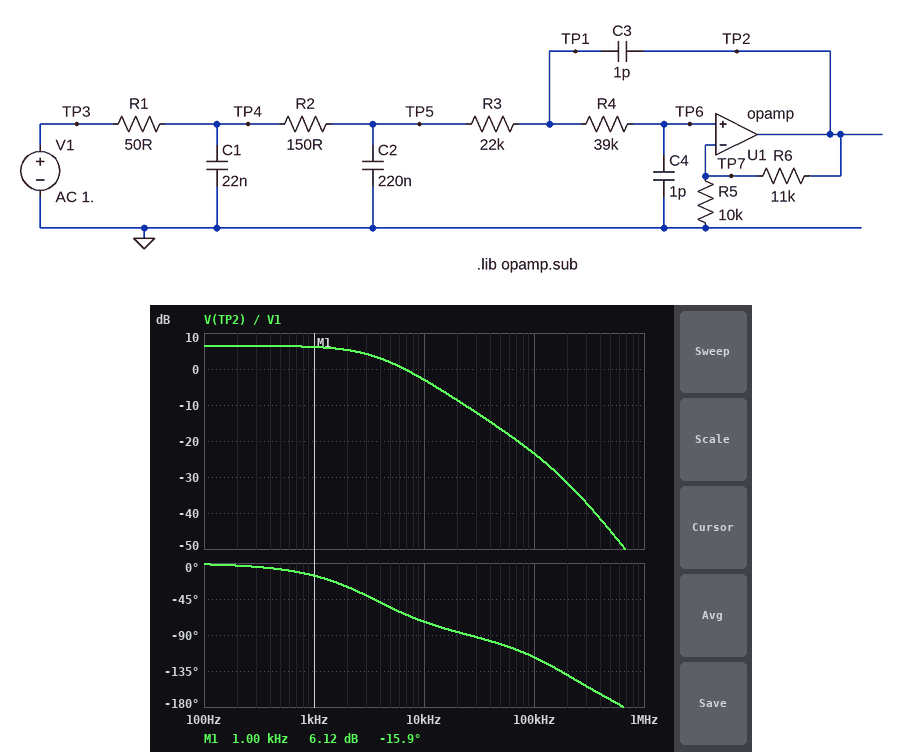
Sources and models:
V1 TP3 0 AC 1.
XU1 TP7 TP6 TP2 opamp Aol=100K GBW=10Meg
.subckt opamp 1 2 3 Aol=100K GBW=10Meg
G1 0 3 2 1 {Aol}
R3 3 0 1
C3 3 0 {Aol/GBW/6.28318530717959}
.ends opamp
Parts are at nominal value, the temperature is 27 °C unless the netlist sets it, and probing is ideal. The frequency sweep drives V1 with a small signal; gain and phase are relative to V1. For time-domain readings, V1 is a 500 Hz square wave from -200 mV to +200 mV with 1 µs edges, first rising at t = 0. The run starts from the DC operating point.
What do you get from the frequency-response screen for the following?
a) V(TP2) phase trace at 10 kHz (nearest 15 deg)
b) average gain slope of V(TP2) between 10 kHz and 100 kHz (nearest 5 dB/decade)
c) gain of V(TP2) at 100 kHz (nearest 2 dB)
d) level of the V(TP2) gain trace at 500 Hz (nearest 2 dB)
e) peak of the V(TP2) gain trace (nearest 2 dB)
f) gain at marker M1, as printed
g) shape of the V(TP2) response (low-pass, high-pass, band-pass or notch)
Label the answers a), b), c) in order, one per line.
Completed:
a) -75 deg
b) -20 dB/decade
c) -24 dB
d) 6 dB
e) 6 dB
f) 6.12 dB
g) low-pass
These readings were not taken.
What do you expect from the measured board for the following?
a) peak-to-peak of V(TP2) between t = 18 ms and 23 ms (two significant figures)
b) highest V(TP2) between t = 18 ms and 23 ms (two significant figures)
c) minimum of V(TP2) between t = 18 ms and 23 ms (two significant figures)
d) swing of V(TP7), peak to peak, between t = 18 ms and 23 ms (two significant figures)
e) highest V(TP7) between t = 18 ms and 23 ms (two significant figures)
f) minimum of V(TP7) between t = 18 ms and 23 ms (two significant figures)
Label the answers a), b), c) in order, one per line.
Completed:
a) 840 mV
b) 420 mV
c) -420 mV
d) 400 mV
e) 200 mV
f) -200 mV
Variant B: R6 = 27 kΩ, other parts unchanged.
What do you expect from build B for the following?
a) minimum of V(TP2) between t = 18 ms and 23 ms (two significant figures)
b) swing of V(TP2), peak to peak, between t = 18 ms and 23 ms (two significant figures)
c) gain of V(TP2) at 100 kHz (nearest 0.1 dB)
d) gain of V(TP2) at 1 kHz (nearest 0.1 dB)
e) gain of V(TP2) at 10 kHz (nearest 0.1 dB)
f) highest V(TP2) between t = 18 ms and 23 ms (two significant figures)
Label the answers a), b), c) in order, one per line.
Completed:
a) -740 mV
b) 1.5 V
c) -18.5 dB
d) 11.0 dB
e) 1.9 dB
f) 740 mV
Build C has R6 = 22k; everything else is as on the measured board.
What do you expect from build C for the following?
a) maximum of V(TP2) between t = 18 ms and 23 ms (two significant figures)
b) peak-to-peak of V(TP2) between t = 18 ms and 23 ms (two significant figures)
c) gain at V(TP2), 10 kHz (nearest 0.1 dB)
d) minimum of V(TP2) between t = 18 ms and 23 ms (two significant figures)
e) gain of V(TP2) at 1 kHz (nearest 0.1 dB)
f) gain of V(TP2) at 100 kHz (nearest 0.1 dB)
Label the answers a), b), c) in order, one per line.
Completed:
a) 640 mV
b) 1.3 V
c) 0.7 dB
d) -640 mV
e) 9.8 dB
f) -19.8 dB
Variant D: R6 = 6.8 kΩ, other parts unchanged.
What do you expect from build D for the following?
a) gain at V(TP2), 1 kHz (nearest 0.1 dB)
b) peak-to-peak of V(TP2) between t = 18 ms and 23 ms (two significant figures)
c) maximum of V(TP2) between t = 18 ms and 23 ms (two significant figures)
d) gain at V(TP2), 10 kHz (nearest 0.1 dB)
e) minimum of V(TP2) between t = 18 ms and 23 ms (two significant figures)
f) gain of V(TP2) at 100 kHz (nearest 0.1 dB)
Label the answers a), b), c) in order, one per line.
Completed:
a) 4.2 dB
b) 670 mV
c) 340 mV
d) -4.9 dB
e) -340 mV
f) -25.4 dB
